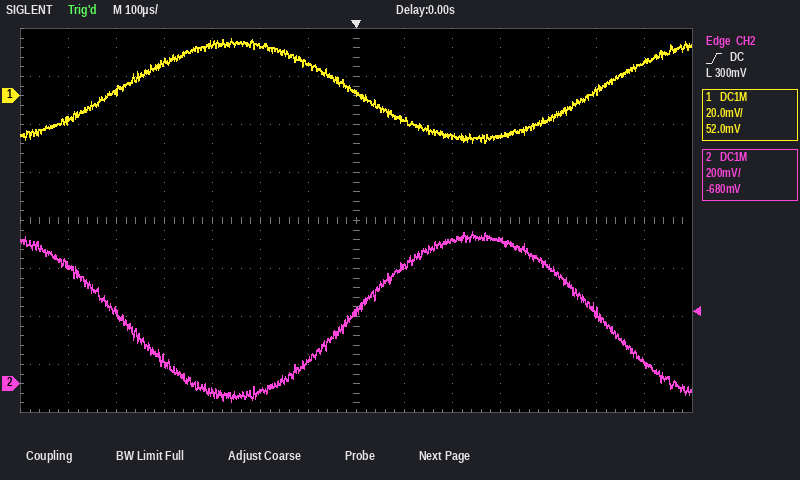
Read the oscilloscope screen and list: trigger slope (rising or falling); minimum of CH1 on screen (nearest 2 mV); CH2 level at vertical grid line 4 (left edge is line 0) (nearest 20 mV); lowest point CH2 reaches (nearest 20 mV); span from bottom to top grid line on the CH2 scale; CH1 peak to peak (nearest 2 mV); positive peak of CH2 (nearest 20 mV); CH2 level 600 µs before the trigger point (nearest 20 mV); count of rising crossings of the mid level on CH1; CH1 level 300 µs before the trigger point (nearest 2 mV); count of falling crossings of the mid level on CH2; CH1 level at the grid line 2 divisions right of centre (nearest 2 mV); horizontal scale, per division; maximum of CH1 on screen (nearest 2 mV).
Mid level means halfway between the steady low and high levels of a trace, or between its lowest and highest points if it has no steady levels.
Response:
rising
-20 mV
-40 mV
-80 mV
1.6 V
44 mV
640 mV
500 mV
2
22 mV
2
-16 mV
100 µs
24 mV
